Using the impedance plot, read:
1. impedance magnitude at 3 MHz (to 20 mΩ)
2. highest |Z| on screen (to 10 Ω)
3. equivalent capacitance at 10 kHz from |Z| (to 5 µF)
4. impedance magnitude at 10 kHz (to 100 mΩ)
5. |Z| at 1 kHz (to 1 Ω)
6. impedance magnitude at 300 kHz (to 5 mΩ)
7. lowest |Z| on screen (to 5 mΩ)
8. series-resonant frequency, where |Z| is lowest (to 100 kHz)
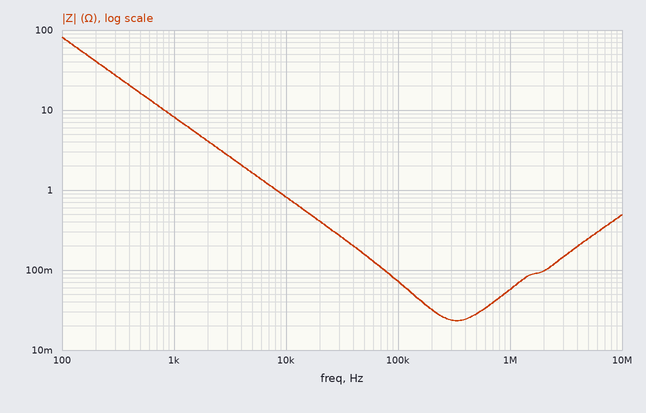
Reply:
140 mΩ
80 Ω
20 µF
800 mΩ
8 Ω
25 mΩ
25 mΩ
300 kHz
